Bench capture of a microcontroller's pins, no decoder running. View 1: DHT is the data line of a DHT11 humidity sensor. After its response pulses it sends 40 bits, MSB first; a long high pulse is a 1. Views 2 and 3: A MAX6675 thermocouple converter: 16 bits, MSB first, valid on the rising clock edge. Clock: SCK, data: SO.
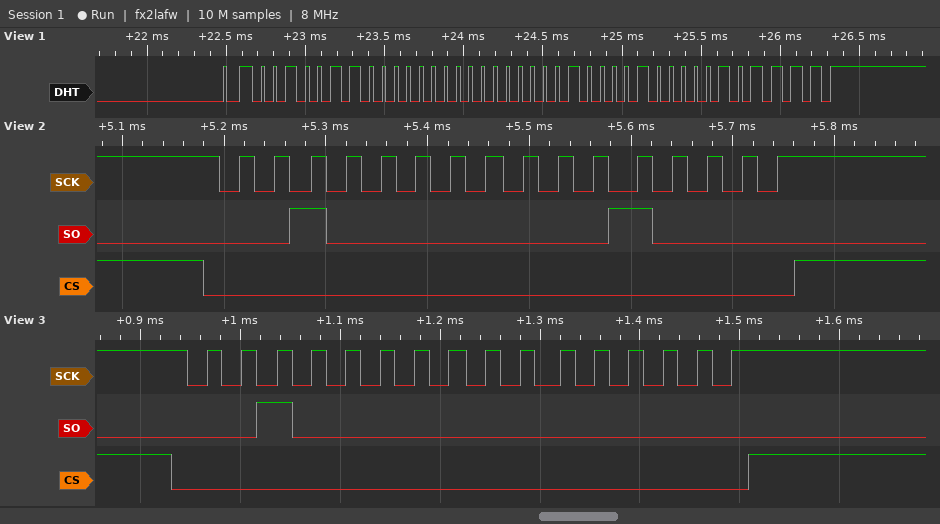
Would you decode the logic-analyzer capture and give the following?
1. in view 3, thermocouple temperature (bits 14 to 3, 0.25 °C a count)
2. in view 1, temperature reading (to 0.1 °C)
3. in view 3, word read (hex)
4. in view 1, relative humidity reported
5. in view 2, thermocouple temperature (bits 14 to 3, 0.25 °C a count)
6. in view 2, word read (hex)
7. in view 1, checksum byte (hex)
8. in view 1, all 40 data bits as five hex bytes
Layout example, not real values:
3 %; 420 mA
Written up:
256.00 °C; 1.8 °C; 0x2000; 38 %; 256.50 °C; 0x2010; 0x2F; 26 00 01 08 2F
